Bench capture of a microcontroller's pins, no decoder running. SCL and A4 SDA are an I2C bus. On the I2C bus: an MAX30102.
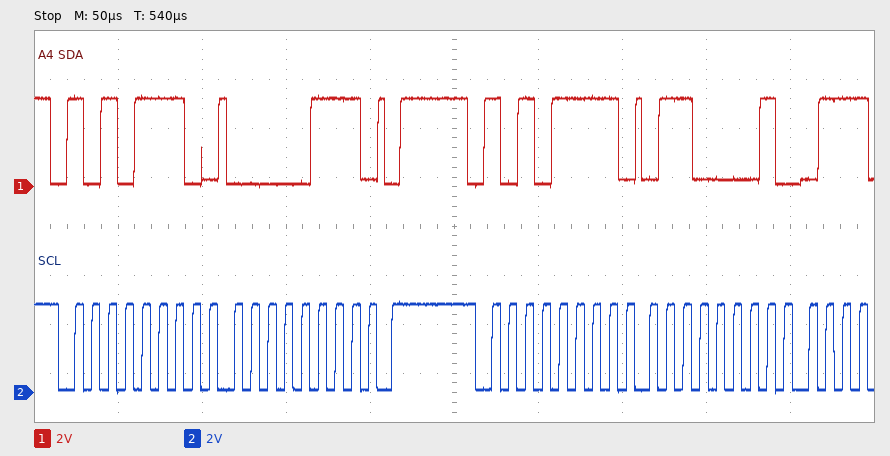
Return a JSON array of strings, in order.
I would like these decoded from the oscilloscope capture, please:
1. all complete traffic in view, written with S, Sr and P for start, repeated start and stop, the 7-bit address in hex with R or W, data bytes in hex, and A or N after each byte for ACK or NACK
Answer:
["S 57W A 07 A P S 57R A 61 A"]
